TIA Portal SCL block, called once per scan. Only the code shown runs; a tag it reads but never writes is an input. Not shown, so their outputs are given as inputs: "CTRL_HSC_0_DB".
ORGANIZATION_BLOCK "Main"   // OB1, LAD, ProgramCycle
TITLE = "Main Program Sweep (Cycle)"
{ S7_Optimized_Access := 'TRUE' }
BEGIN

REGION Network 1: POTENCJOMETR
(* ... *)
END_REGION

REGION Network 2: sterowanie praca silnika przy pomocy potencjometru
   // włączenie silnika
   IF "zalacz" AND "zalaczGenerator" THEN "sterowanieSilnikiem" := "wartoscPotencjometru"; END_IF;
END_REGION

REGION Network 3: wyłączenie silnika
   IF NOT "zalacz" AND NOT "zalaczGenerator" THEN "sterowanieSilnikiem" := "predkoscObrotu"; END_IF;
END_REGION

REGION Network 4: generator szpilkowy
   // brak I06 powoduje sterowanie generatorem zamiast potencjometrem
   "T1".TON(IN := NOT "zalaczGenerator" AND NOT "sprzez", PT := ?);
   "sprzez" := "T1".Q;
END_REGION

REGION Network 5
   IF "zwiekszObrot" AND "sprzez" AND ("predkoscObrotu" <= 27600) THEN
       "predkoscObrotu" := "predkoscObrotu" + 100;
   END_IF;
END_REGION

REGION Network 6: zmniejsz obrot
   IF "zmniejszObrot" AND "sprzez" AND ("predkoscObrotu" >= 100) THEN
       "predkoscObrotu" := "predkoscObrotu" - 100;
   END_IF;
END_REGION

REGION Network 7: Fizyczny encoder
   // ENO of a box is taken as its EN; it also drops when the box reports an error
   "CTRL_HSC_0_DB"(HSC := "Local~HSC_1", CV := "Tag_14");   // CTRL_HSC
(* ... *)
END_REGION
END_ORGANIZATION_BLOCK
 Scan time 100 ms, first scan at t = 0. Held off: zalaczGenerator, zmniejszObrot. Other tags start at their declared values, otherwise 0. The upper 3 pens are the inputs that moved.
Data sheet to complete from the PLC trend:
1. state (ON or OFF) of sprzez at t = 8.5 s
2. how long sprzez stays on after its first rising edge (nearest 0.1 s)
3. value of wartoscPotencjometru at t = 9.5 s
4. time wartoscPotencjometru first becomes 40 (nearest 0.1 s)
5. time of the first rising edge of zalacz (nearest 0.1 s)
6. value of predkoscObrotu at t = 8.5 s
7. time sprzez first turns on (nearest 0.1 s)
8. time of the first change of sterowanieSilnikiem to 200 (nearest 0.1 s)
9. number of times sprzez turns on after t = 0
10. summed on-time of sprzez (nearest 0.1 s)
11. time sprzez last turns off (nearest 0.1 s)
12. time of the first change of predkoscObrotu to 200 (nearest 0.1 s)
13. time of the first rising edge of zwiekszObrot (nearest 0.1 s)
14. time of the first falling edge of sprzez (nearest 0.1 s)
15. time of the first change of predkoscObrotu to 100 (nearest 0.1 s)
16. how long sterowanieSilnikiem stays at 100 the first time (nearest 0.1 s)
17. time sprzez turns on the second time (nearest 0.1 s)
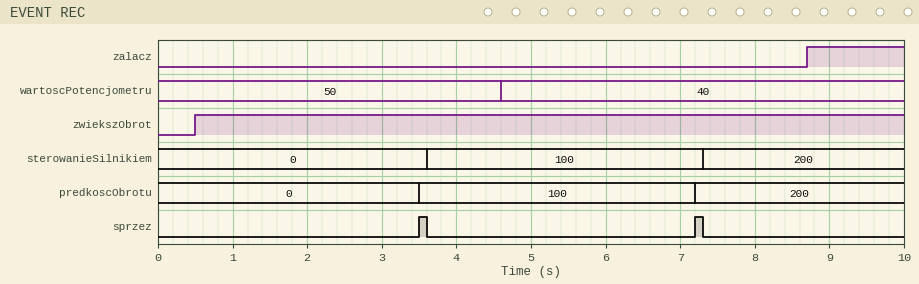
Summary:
OFF
0.1 s
40
4.6 s
8.7 s
200
3.5 s
7.3 s
2
0.2 s
7.3 s
7.2 s
0.5 s
3.6 s
3.5 s
3.7 s
7.2 s
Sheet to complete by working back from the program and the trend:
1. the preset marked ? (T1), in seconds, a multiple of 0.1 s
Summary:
3.5 s
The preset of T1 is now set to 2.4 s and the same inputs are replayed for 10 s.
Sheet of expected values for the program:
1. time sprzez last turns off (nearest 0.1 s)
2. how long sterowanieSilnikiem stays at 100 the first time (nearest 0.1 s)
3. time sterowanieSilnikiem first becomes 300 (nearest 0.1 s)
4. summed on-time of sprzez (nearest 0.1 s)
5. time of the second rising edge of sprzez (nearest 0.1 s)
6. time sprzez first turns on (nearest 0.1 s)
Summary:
7.7 s
2.6 s
7.7 s
0.3 s
5.0 s
2.4 s
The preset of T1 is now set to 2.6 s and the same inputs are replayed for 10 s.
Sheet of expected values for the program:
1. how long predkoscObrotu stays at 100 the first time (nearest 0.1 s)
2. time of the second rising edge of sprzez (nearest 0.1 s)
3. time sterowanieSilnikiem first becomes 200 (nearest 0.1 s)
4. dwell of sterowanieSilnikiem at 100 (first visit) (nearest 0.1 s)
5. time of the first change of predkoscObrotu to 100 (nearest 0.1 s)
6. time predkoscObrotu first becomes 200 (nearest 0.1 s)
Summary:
2.8 s
5.4 s
5.5 s
2.8 s
2.6 s
5.4 s
